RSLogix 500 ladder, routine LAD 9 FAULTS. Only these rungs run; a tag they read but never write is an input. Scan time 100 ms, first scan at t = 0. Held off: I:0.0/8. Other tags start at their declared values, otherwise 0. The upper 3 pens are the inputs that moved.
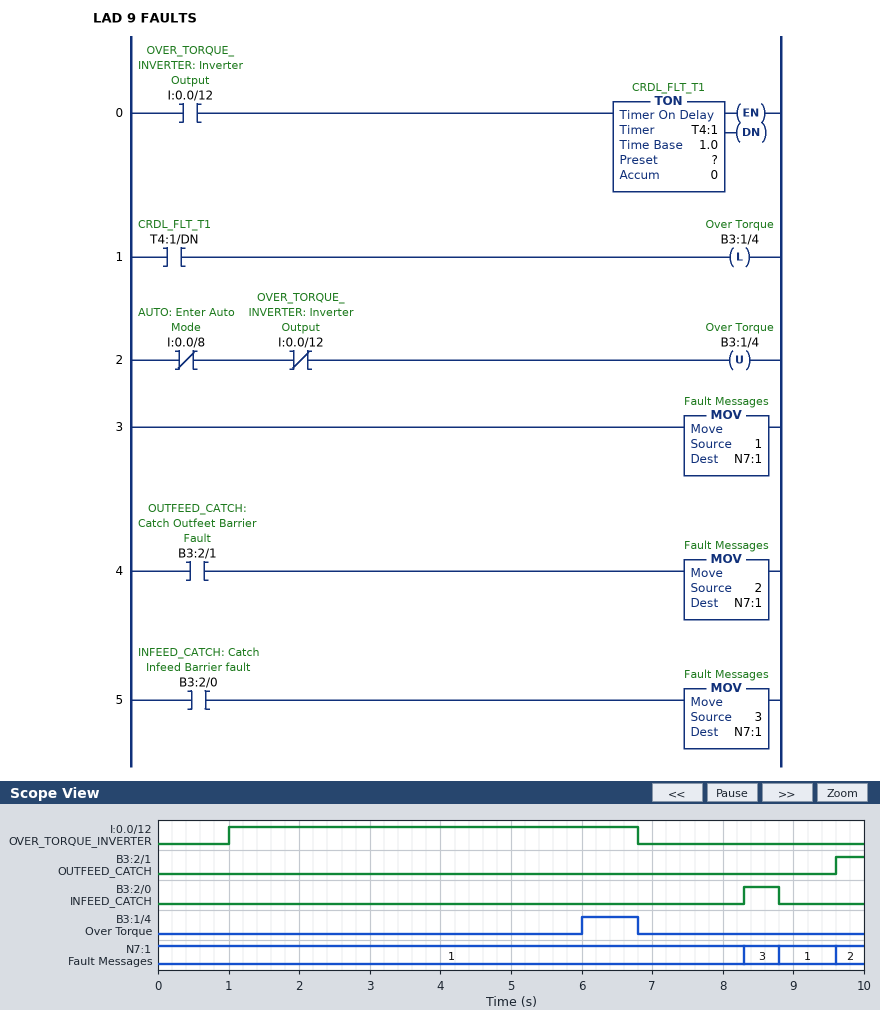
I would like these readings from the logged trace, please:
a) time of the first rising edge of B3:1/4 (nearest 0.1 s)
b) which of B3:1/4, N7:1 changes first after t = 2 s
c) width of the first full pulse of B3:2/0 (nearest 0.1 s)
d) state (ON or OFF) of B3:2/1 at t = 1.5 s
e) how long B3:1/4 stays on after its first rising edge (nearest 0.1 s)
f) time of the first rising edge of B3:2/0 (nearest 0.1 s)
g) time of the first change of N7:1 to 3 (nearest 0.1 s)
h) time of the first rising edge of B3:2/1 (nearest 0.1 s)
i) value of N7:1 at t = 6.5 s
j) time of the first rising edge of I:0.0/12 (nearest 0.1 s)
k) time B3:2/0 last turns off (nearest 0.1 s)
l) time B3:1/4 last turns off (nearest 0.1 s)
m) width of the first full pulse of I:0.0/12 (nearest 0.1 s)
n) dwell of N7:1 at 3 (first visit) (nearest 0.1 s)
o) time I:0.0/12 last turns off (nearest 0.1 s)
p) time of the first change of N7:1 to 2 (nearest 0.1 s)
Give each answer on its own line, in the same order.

6.0 s
B3:1/4
0.5 s
OFF
0.8 s
8.3 s
8.3 s
9.6 s
1
1.0 s
8.8 s
6.8 s
5.8 s
0.5 s
6.8 s
9.6 s
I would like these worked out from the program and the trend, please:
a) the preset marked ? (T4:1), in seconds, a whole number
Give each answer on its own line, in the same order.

5 s
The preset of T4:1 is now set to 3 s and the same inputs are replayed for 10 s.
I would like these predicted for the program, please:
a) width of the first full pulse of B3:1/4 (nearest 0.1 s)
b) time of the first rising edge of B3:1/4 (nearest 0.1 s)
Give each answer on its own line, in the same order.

2.8 s
4.0 s
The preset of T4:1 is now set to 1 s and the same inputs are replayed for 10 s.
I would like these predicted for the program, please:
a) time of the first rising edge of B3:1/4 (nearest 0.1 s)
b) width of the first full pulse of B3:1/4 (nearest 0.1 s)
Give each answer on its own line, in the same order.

2.0 s
4.8 s
